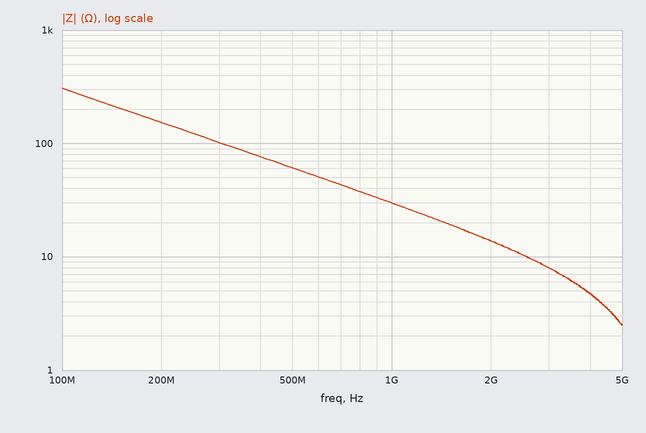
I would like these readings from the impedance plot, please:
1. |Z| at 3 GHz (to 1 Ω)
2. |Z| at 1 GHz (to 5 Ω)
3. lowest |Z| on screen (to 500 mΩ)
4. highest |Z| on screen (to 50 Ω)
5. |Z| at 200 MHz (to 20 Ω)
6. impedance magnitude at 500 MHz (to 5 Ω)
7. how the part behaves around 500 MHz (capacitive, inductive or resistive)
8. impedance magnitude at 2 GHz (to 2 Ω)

8 Ω
30 Ω
2.5 Ω
300 Ω
160 Ω
60 Ω
capacitive
14 Ω
